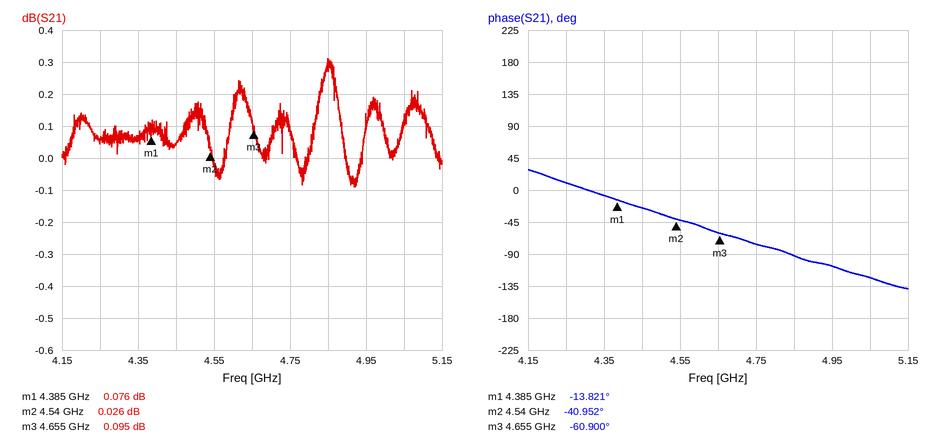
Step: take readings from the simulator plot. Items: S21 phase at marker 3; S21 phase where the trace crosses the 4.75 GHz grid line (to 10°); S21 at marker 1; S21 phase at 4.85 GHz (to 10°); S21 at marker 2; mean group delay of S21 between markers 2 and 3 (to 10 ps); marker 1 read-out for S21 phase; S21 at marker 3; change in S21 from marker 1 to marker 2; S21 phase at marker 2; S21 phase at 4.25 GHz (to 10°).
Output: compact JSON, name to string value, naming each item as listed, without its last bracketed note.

{"S21 phase at marker 3": "-60.900°", "S21 phase where the trace crosses the 4.75 GHz grid line": "-80°", "S21 at marker 1": "0.076 dB", "S21 phase at 4.85 GHz": "-90°", "S21 at marker 2": "0.026 dB", "mean group delay of S21 between markers 2 and 3": "480 ps", "marker 1 read-out for S21 phase": "-13.821°", "S21 at marker 3": "0.095 dB", "change in S21 from marker 1 to marker 2": "-0.050 dB", "S21 phase at marker 2": "-40.952°", "S21 phase at 4.25 GHz": "10°"}
